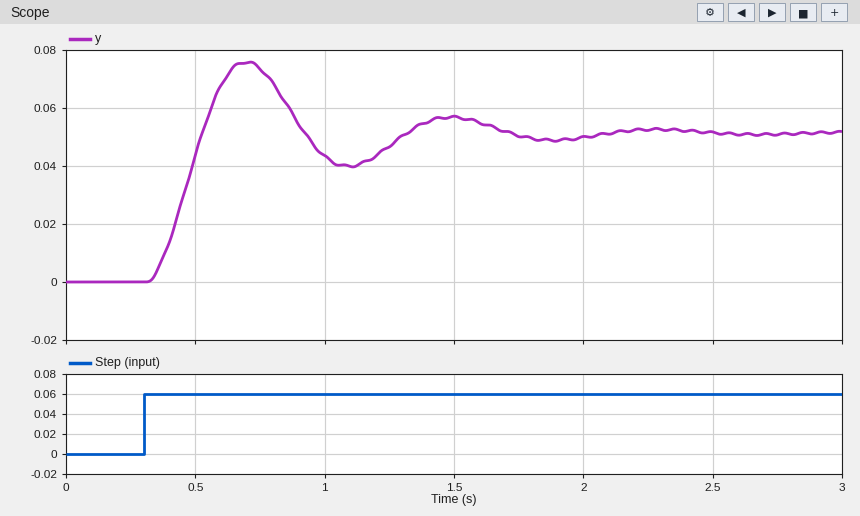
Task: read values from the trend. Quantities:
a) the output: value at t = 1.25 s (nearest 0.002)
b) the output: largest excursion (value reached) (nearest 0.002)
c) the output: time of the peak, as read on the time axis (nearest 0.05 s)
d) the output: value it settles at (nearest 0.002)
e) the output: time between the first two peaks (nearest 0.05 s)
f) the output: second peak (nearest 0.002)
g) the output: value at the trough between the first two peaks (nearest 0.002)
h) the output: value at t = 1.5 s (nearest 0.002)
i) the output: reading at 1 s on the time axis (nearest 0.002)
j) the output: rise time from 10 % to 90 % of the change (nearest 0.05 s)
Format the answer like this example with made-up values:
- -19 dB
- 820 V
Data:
- 0.046
- 0.076
- 0.70 s
- 0.052
- 0.80 s
- 0.058
- 0.040
- 0.058
- 0.044
- 0.15 s
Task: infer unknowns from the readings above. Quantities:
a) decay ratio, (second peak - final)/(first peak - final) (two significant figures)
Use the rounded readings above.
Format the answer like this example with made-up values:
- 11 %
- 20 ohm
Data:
- 0.25
